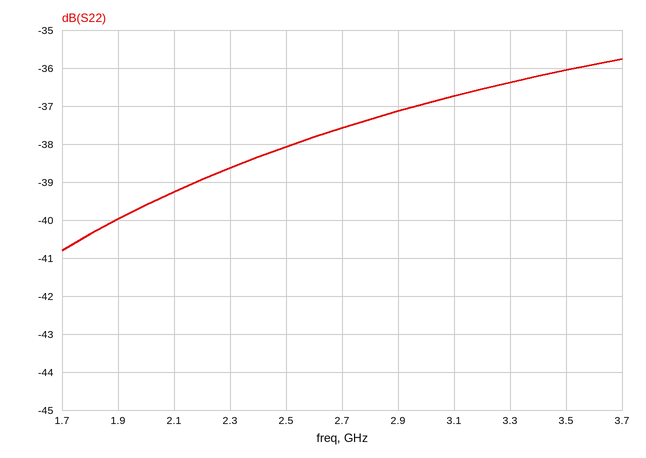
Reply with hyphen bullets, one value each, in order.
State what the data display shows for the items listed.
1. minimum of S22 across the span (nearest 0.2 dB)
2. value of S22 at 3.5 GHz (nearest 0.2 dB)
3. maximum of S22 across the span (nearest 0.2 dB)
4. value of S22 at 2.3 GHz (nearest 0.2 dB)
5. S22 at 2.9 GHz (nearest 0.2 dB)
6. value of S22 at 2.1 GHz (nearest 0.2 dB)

- -40.8 dB
- -36.0 dB
- -35.8 dB
- -38.6 dB
- -37.2 dB
- -39.2 dB
